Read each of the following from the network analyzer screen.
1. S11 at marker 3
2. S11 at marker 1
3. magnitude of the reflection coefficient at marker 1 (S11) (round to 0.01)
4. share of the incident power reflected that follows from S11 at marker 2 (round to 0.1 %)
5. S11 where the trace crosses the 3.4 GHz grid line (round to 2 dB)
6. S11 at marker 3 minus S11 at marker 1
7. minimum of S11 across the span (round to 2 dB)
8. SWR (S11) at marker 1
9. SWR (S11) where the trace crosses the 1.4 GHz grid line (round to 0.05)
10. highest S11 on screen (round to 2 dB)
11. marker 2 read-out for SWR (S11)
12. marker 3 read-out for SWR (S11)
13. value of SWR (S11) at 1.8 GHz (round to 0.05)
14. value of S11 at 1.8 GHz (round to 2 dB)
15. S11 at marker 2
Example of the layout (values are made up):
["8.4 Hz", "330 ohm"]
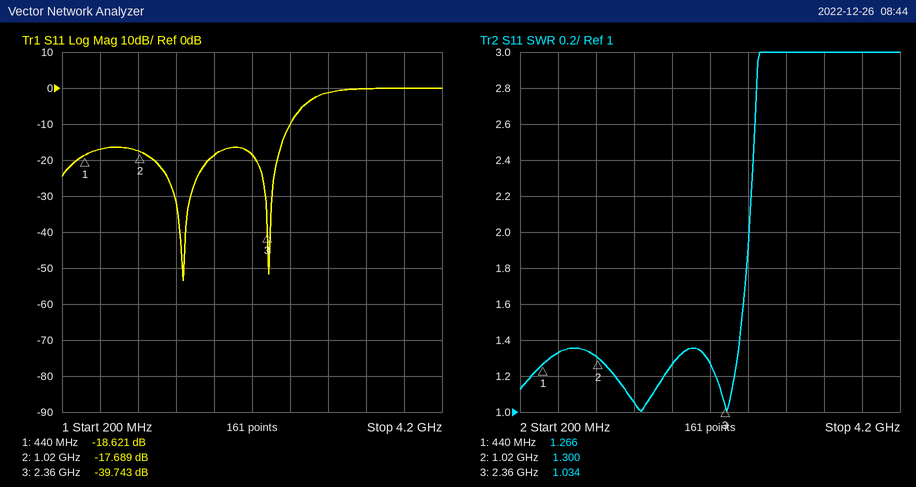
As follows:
["-39.743 dB", "-18.621 dB", "0.12", "1.7 %", "0 dB", "-21.122 dB", "-54 dB", "1.266", "1.05", "0 dB", "1.300", "1.034", "1.25", "-18 dB", "-17.689 dB"]
